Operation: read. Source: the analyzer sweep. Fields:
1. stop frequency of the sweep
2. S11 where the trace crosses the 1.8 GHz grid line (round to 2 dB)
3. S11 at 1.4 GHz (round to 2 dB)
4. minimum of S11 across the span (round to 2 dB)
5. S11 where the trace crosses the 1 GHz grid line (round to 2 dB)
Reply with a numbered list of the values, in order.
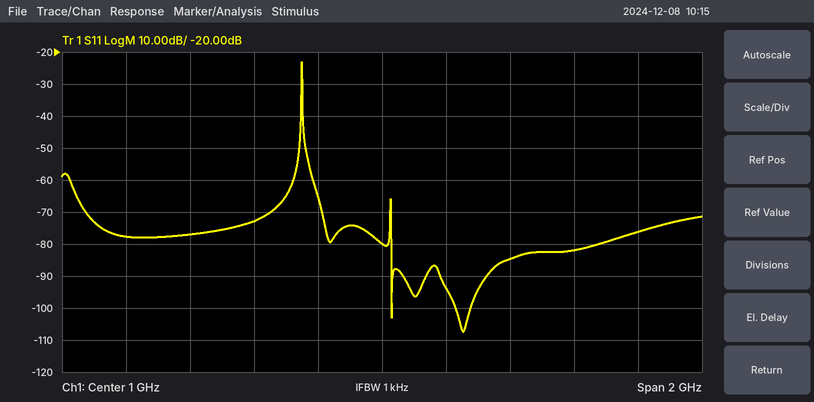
1. 2 GHz
2. -76 dB
3. -84 dB
4. -108 dB
5. -80 dB
